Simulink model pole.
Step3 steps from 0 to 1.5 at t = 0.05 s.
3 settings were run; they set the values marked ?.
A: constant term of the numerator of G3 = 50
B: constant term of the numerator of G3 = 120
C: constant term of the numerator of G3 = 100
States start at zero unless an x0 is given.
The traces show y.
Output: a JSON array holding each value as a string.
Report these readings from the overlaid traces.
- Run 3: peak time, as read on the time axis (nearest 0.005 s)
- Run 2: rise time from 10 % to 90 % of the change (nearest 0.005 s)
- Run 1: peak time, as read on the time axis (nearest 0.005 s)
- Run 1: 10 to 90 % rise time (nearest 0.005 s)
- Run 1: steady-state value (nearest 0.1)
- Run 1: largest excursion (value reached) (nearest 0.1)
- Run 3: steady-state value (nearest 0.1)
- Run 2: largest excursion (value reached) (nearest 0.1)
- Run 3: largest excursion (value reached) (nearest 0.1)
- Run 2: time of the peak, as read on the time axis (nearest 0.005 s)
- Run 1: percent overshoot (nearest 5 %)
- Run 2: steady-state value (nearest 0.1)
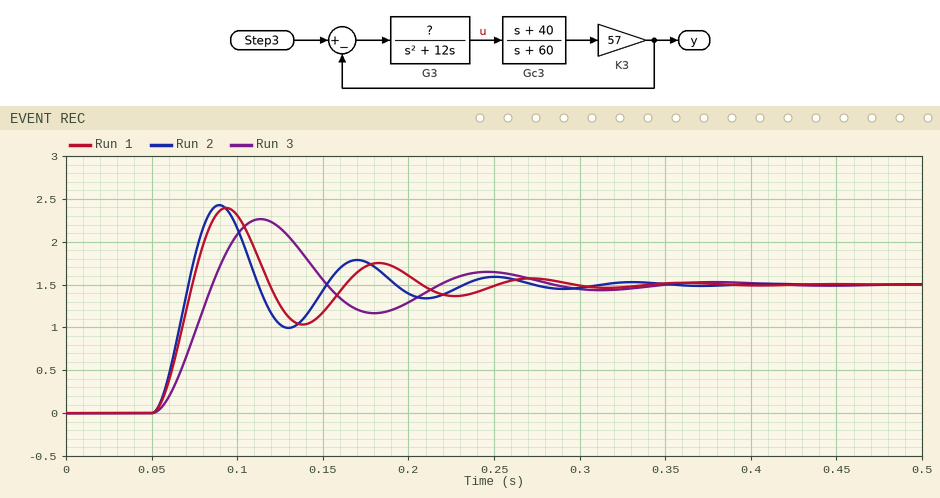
["0.115 s", "0.015 s", "0.095 s", "0.015 s", "1.5", "2.4", "1.5", "2.4", "2.3", "0.090 s", "60 %", "1.5"]
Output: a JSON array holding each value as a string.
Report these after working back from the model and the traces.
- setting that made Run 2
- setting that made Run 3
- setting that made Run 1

["B", "A", "C"]
